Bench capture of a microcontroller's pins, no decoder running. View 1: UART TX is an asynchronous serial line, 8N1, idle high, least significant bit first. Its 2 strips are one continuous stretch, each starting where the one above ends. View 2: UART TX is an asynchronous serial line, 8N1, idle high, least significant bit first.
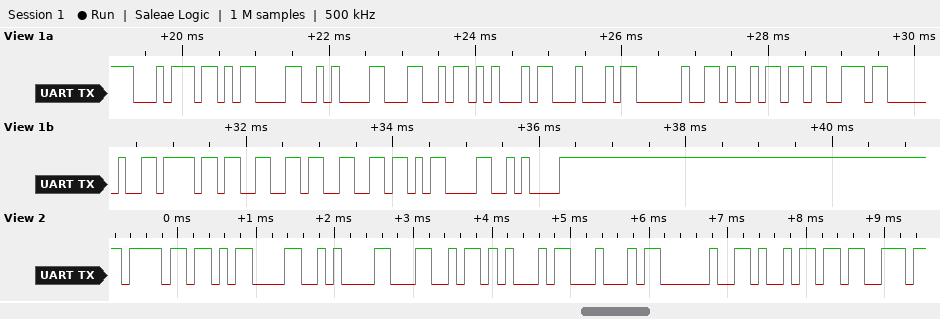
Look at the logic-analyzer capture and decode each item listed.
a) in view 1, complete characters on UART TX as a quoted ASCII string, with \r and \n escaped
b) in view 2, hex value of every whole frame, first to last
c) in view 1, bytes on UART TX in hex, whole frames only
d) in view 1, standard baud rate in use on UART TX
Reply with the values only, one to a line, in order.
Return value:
"t\r\nLED is off\r\n"
6F 0D 0A 4C 45 44 20 69 73
0x74 0x0D 0x0A 0x4C 0x45 0x44 0x20 0x69 0x73 0x20 0x6F 0x66 0x66 0x0D 0x0A
9600 baud
